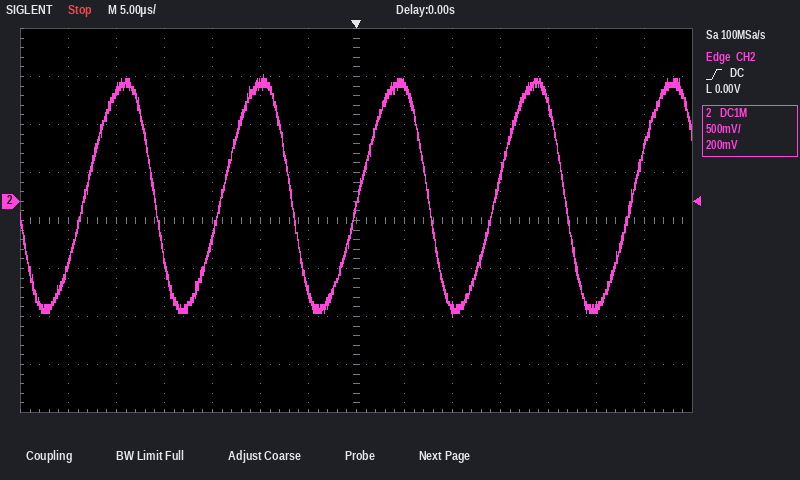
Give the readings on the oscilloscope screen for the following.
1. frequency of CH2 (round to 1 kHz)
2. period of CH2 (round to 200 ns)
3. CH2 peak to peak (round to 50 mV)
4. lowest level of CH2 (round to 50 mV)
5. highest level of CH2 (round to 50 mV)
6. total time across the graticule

70 kHz
14.2 µs
2.50 V
-1.20 V
1.30 V
70 µs
